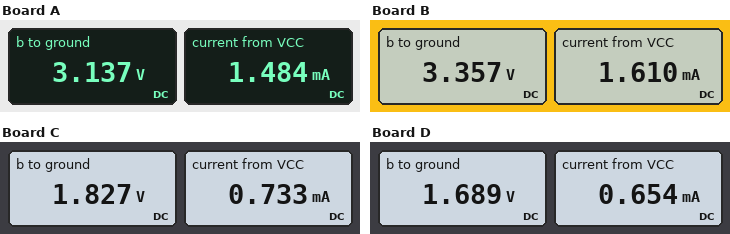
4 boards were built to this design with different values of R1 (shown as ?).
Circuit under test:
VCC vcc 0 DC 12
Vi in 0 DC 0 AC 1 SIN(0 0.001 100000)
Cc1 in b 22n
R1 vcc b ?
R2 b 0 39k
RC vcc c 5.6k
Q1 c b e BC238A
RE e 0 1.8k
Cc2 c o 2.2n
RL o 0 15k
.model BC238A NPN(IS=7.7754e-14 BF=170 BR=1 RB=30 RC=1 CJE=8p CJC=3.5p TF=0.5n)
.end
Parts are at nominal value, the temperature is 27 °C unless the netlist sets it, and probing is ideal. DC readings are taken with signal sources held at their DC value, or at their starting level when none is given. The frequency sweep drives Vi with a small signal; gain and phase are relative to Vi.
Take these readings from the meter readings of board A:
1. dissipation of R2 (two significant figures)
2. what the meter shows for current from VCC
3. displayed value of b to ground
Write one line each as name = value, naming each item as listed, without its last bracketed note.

dissipation of R2 = 250 µW
what the meter shows for current from VCC = 1.484 mA
displayed value of b to ground = 3.137 V
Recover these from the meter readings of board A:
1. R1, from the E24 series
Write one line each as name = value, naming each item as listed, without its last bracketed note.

R1, from the E24 series = 100 kΩ
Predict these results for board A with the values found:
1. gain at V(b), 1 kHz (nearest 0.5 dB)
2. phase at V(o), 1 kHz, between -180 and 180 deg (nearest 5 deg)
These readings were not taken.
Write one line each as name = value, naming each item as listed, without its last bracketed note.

gain at V(b), 1 kHz = -0.5 dB
phase at V(o), 1 kHz, between -180 and 180 deg = -90 deg
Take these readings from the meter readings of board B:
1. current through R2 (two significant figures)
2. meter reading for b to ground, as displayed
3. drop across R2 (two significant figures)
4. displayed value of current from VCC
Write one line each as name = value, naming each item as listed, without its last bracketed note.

current through R2 = 86 µA
meter reading for b to ground, as displayed = 3.357 V
drop across R2 = 3.4 V
displayed value of current from VCC = 1.610 mA
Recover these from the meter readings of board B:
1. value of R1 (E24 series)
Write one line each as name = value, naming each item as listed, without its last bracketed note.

value of R1 = 91 kΩ
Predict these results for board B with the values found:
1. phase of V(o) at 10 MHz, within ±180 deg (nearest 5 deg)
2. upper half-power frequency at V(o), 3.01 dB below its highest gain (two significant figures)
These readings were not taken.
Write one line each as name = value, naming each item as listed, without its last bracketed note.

phase of V(o) at 10 MHz, within ±180 deg = 115 deg
upper half-power frequency at V(o), 3.01 dB below its highest gain = 16 MHz
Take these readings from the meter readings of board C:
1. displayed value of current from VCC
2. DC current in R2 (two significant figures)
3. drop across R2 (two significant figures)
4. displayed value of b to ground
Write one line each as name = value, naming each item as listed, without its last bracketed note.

displayed value of current from VCC = 0.733 mA
DC current in R2 = 47 µA
drop across R2 = 1.8 V
displayed value of b to ground = 1.827 V
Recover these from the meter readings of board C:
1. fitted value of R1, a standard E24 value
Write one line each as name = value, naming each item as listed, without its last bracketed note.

fitted value of R1, a standard E24 value = 200 kΩ
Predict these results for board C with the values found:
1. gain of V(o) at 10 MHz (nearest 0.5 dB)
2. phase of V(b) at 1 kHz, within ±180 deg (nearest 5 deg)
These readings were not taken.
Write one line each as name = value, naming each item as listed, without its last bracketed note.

gain of V(o) at 10 MHz = 6.5 dB
phase of V(b) at 1 kHz, within ±180 deg = 15 deg
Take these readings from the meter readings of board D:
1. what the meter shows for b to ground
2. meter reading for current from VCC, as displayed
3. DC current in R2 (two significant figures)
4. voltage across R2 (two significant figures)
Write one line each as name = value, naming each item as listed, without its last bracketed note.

what the meter shows for b to ground = 1.689 V
meter reading for current from VCC, as displayed = 0.654 mA
DC current in R2 = 43 µA
voltage across R2 = 1.7 V
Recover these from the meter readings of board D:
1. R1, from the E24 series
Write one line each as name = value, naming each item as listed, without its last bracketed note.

R1, from the E24 series = 220 kΩ
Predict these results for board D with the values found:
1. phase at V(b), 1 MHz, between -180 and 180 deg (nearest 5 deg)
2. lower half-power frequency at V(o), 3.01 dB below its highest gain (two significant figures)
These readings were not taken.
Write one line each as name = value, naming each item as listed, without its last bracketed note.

phase at V(b), 1 MHz, between -180 and 180 deg = 0 deg
lower half-power frequency at V(o), 3.01 dB below its highest gain = 3.5 kHz
